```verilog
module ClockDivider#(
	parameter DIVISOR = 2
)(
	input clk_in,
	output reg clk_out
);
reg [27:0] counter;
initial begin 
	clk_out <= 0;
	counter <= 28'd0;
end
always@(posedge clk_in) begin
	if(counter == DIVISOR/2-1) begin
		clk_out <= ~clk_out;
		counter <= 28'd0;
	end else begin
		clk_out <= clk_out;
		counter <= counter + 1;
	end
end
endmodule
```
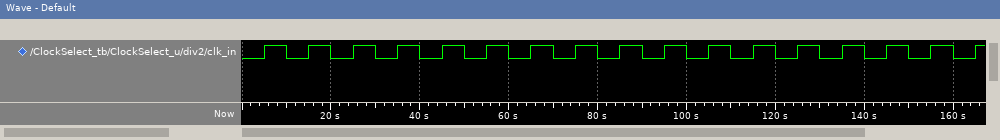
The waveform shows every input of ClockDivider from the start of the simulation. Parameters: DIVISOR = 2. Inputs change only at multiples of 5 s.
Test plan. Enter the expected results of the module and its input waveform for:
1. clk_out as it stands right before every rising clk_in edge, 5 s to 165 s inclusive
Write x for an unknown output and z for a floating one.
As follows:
0 1 0 1 0 1 0 1 0 1 0 1 0 1 0 1 0
